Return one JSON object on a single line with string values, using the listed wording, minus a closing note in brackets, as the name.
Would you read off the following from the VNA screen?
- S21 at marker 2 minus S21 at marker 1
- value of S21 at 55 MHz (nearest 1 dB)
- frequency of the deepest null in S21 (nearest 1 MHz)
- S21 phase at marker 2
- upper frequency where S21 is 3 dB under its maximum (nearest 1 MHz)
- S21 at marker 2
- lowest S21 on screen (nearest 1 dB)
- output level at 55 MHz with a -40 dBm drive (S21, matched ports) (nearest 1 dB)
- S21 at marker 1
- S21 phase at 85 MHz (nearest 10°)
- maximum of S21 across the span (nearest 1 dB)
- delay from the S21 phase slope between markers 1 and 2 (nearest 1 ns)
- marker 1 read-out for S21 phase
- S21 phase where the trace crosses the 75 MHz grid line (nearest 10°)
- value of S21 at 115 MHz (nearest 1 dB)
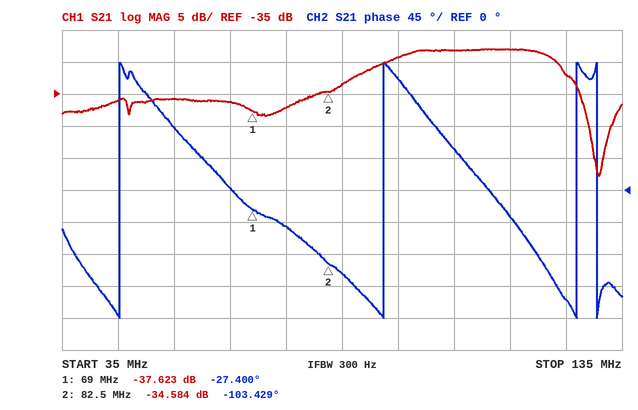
{"S21 at marker 2 minus S21 at marker 1": "3.039 dB", "value of S21 at 55 MHz": "-36 dB", "frequency of the deepest null in S21": "131 MHz", "S21 phase at marker 2": "-103.429°", "upper frequency where S21 is 3 dB under its maximum": "124 MHz", "S21 at marker 2": "-34.584 dB", "lowest S21 on screen": "-48 dB", "output level at 55 MHz with a -40 dBm drive (S21, matched ports)": "-76 dBm", "S21 at marker 1": "-37.623 dB", "S21 phase at 85 MHz": "-120°", "maximum of S21 across the span": "-28 dB", "delay from the S21 phase slope between markers 1 and 2": "16 ns", "marker 1 read-out for S21 phase": "-27.400°", "S21 phase where the trace crosses the 75 MHz grid line": "-50°", "value of S21 at 115 MHz": "-28 dB"}
